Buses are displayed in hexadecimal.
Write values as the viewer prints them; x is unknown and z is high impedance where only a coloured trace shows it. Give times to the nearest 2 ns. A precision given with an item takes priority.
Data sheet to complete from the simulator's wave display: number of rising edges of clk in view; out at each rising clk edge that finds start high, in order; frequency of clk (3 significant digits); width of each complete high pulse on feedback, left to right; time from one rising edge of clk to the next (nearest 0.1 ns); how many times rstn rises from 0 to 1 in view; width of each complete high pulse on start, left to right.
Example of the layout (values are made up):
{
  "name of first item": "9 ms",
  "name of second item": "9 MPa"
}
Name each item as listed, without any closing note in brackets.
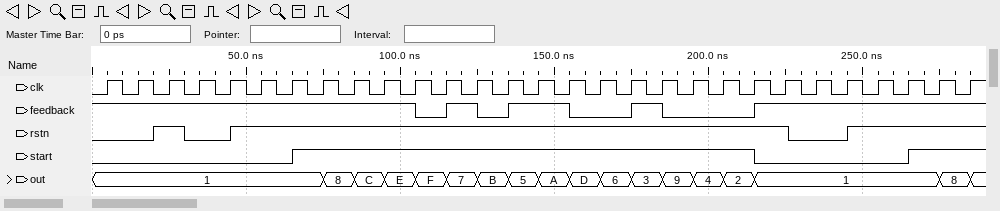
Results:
{
  "number of rising edges of clk in view": "29",
  "out at each rising clk edge that finds start high, in order": "1, 8, C, E, F, 7, B, 5, A, D, 6, 3, 9, 4, 2, 1, 8",
  "frequency of clk": "100 MHz",
  "width of each complete high pulse on feedback, left to right": "10 ns, 20 ns, 10 ns",
  "time from one rising edge of clk to the next": "10 ns",
  "how many times rstn rises from 0 to 1 in view": "3",
  "width of each complete high pulse on start, left to right": "150 ns"
}
